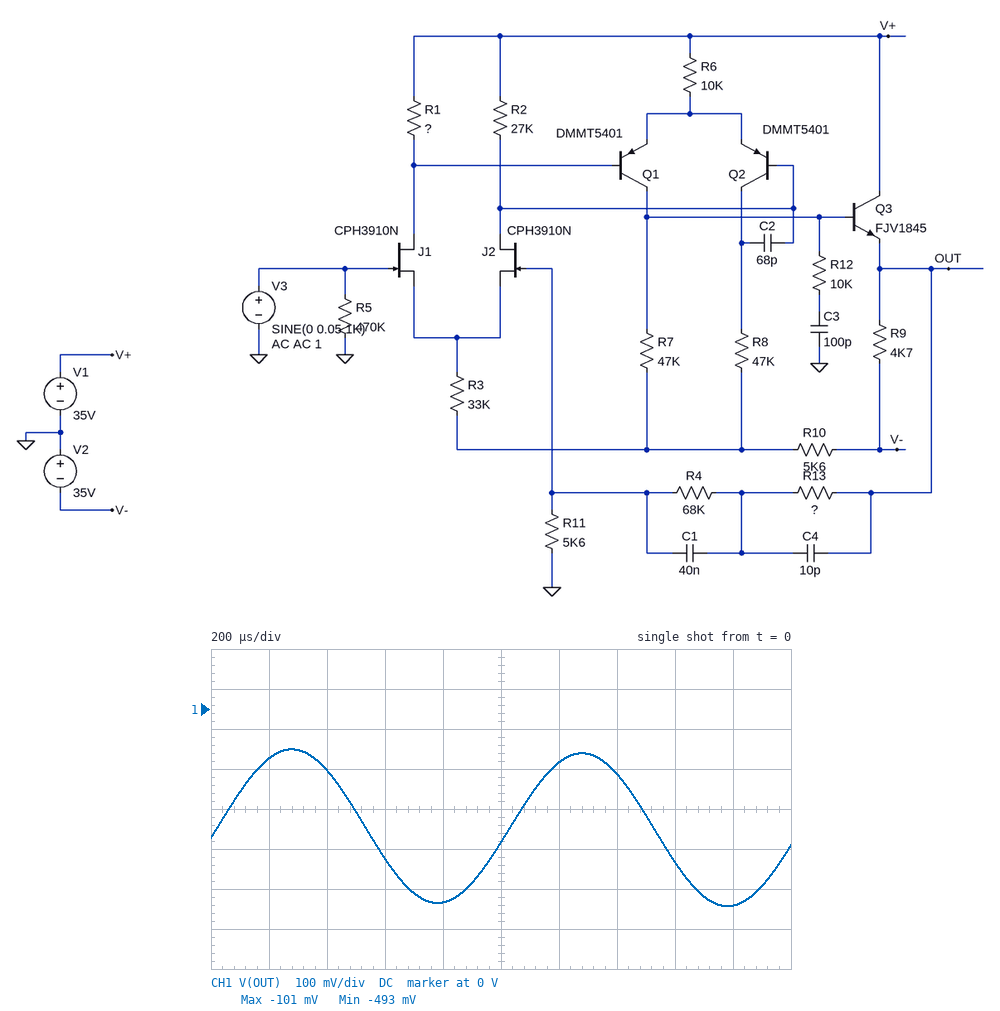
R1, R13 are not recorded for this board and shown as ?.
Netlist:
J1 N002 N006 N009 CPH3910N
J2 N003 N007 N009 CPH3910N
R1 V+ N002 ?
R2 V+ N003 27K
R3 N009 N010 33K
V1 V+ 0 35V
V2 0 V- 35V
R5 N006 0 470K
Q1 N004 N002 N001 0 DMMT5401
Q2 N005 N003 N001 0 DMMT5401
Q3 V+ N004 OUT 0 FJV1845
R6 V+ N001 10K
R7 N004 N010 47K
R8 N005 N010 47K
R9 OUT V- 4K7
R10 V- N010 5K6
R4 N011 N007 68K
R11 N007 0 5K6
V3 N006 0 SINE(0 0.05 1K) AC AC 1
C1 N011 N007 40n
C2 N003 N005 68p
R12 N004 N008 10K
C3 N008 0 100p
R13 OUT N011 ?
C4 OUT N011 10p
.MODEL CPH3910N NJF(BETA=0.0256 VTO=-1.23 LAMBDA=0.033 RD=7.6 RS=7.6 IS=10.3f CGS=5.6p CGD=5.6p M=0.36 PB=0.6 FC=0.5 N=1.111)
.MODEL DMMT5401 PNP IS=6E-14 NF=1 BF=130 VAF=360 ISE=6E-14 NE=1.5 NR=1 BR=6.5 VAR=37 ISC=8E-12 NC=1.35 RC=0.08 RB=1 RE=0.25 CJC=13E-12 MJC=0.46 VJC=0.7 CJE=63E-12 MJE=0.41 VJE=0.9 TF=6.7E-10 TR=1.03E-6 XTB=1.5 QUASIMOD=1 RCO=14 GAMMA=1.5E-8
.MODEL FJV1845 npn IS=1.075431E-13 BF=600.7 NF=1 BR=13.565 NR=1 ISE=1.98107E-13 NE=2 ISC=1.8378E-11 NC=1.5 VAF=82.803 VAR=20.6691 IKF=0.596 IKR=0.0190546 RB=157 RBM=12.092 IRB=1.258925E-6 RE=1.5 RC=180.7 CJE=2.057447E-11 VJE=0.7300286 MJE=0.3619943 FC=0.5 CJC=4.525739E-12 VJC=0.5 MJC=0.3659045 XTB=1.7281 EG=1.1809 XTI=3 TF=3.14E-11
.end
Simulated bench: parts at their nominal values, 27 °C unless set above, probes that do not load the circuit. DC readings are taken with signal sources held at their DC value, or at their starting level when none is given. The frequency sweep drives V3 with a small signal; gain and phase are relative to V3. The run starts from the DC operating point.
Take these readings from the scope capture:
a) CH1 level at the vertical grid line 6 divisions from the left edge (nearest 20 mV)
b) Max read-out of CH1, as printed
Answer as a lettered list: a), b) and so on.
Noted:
a) -140 mV
b) -101 mV
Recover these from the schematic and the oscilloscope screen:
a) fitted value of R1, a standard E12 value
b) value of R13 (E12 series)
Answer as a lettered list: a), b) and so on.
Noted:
a) 18 kΩ
b) 15 kΩ
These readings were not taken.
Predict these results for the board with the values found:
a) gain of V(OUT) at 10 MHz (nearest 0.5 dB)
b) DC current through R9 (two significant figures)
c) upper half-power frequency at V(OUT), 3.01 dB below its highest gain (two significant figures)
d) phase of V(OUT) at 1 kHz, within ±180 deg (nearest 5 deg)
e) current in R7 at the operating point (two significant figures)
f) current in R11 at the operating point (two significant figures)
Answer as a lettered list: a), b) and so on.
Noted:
a) 1.5 dB
b) 7.4 mA
c) 62 Hz
d) -10 deg
e) 560 µA
f) 3.6 µA
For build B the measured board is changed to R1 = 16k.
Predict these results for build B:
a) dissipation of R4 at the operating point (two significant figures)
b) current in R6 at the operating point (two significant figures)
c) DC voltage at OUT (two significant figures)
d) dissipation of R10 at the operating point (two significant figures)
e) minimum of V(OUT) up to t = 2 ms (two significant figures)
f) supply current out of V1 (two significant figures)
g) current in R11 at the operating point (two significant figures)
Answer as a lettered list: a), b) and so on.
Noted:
a) 1.5 µW
b) 770 µA
c) -410 mV
d) 14 mW
e) -580 mV
f) 8.9 mA
g) 4.7 µA
